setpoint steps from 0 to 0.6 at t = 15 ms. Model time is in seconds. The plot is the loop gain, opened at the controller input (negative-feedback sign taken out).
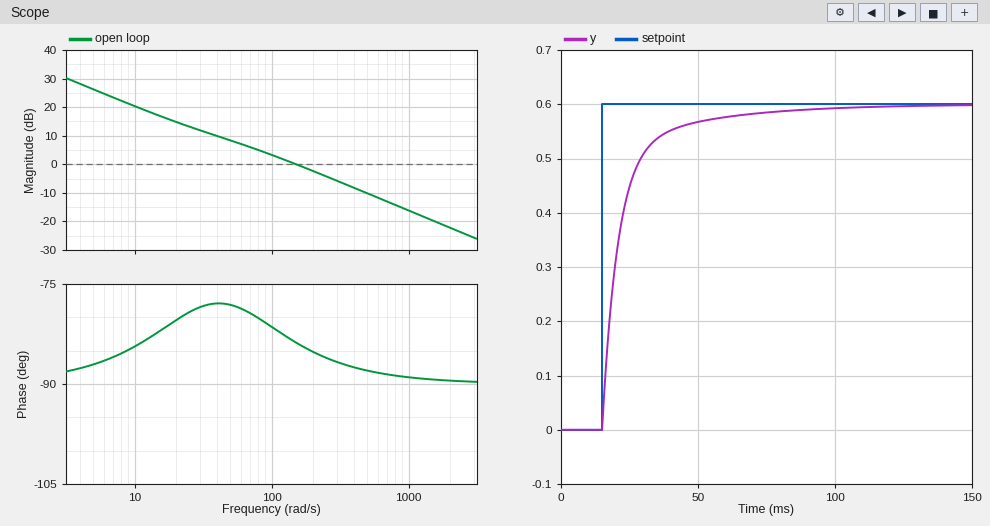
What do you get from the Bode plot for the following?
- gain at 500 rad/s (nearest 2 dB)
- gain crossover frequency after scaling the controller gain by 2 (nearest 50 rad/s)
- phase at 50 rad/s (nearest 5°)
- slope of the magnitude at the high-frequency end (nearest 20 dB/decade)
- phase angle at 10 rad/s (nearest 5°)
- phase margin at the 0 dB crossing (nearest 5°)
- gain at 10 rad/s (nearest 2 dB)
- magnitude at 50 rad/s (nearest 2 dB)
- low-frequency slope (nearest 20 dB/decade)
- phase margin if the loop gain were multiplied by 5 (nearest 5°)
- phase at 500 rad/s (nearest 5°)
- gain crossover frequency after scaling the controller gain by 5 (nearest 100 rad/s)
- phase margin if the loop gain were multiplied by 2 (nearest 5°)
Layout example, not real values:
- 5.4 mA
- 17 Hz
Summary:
- -10 dB
- 300 rad/s
- -80°
- -20 dB/decade
- -85°
- 95°
- 20 dB
- 8 dB
- -20 dB/decade
- 90°
- -90°
- 800 rad/s
- 95°
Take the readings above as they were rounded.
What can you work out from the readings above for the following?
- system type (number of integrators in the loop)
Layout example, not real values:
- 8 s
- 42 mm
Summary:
- 1
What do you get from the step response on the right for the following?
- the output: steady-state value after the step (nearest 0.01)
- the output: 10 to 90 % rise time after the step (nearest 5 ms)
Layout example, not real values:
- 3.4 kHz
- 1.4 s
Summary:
- 0.60
- 20 ms
